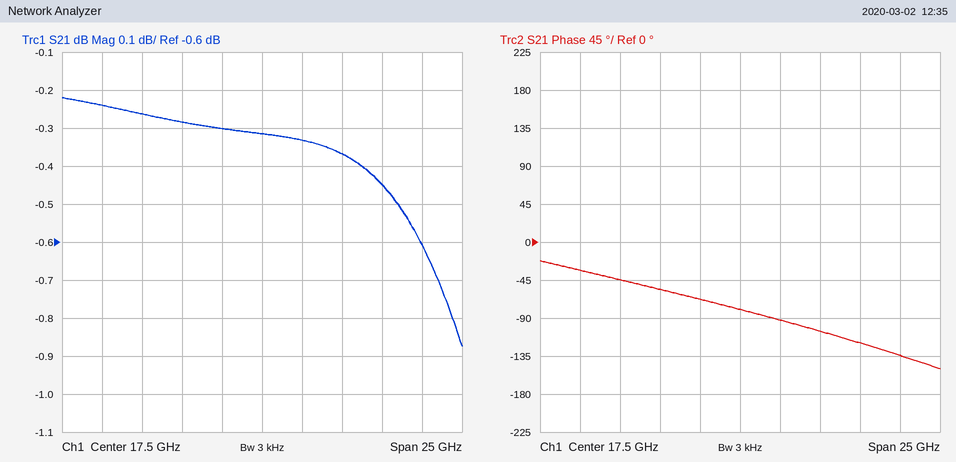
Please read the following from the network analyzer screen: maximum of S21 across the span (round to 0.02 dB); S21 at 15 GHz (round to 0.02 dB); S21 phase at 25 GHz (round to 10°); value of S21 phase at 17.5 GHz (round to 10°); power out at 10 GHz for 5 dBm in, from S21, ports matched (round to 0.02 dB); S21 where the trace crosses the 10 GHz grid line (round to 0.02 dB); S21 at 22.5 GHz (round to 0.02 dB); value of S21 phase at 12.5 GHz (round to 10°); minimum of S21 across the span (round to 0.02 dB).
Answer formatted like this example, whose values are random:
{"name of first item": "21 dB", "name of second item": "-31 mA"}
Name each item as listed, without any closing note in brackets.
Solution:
{"maximum of S21 across the span": "-0.22 dB", "S21 at 15 GHz": "-0.30 dB", "S21 phase at 25 GHz": "-120°", "value of S21 phase at 17.5 GHz": "-80°", "power out at 10 GHz for 5 dBm in, from S21, ports matched": "4.74 dBm", "S21 where the trace crosses the 10 GHz grid line": "-0.26 dB", "S21 at 22.5 GHz": "-0.36 dB", "value of S21 phase at 12.5 GHz": "-60°", "minimum of S21 across the span": "-0.88 dB"}
